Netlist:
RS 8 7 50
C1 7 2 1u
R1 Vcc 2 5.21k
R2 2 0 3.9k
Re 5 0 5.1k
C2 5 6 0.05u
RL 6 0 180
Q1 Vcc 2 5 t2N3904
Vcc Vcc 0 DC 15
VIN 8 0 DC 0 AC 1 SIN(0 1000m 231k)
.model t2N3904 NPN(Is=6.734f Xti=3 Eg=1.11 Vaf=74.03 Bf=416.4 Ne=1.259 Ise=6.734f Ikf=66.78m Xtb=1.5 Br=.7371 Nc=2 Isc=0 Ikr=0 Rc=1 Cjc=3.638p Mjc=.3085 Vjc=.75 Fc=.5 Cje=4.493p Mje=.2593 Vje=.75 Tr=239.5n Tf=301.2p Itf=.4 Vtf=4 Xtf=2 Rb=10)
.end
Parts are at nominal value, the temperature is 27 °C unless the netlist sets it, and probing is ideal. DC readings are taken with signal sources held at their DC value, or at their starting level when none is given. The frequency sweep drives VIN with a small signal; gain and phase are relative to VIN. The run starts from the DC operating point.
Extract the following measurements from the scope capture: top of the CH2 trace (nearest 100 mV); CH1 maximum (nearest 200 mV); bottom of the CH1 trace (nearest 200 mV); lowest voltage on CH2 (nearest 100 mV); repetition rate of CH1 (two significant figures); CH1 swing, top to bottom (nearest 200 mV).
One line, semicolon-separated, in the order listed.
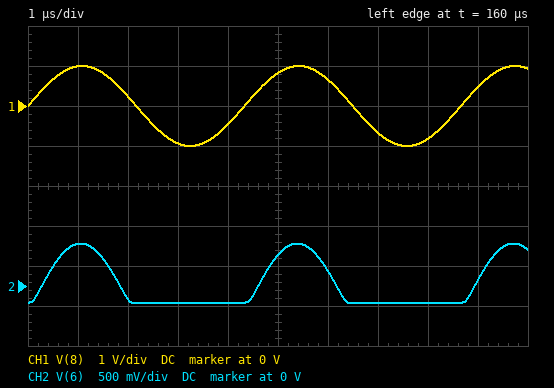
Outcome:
500 mV; 1.0 V; -1.0 V; -200 mV; 230 kHz; 2.0 V
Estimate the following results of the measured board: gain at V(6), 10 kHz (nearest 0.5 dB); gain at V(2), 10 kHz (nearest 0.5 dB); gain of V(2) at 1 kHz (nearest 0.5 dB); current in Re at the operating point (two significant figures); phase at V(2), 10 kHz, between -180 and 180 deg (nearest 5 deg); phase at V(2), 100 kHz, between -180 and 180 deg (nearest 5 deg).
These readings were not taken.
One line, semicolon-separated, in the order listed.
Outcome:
-6.5 dB; 0 dB; 0 dB; 1.1 mA; 0 deg; 0 deg
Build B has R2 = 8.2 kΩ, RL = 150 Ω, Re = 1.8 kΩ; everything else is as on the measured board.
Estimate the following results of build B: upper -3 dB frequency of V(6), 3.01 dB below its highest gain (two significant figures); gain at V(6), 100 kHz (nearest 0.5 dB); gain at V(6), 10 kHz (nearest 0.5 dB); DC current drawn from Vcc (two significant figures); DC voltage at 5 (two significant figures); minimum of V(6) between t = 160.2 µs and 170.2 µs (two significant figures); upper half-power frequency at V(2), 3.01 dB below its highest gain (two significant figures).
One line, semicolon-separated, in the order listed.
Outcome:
690 MHz; -0.5 dB; -7.5 dB; 5.8 mA; 8.4 V; -650 mV; 770 MHz
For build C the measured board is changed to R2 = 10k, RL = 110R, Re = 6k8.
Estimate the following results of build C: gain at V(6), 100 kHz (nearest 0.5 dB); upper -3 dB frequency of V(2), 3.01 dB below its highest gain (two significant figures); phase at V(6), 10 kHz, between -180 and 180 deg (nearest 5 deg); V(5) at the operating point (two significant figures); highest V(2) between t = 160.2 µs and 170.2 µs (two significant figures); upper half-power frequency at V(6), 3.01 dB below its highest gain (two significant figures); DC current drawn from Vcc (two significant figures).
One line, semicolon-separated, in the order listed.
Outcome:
-2.0 dB; 570 MHz; 70 deg; 9.2 V; 11 V; 750 MHz; 2.3 mA
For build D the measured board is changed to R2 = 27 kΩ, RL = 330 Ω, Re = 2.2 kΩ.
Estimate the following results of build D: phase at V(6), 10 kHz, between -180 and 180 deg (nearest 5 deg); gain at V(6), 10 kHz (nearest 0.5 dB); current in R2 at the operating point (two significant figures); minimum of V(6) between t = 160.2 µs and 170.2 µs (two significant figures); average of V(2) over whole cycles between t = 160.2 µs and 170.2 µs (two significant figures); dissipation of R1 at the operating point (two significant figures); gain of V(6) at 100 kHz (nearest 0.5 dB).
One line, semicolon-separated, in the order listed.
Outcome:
45 deg; -3.0 dB; 460 µA; -960 mV; 12 V; 1.3 mW; -0.5 dB
